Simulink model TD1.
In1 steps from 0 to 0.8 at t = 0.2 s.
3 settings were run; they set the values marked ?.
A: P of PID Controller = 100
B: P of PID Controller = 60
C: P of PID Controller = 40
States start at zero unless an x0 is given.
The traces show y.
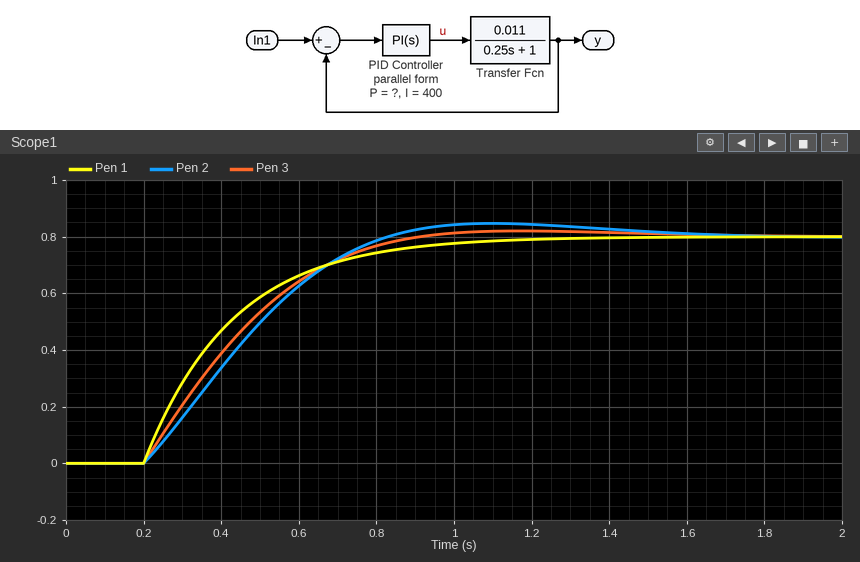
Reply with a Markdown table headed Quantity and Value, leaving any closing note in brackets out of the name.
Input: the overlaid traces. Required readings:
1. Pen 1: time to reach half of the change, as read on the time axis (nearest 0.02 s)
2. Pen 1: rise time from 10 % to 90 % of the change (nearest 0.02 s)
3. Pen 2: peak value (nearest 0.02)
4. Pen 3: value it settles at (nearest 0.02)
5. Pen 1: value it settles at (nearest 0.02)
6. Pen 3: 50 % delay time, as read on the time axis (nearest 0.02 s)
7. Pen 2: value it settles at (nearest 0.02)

| Quantity | Value |
|---|---|
| Pen 1: time to reach half of the change, as read on the time axis | 0.36 s |
| Pen 1: rise time from 10 % to 90 % of the change | 0.50 s |
| Pen 2: peak value | 0.84 |
| Pen 3: value it settles at | 0.80 |
| Pen 1: value it settles at | 0.80 |
| Pen 3: 50 % delay time, as read on the time axis | 0.40 s |
| Pen 2: value it settles at | 0.80 |
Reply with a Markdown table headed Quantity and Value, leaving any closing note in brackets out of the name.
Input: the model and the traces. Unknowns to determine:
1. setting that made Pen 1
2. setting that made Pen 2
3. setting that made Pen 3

| Quantity | Value |
|---|---|
| setting that made Pen 1 | A |
| setting that made Pen 2 | C |
| setting that made Pen 3 | B |
